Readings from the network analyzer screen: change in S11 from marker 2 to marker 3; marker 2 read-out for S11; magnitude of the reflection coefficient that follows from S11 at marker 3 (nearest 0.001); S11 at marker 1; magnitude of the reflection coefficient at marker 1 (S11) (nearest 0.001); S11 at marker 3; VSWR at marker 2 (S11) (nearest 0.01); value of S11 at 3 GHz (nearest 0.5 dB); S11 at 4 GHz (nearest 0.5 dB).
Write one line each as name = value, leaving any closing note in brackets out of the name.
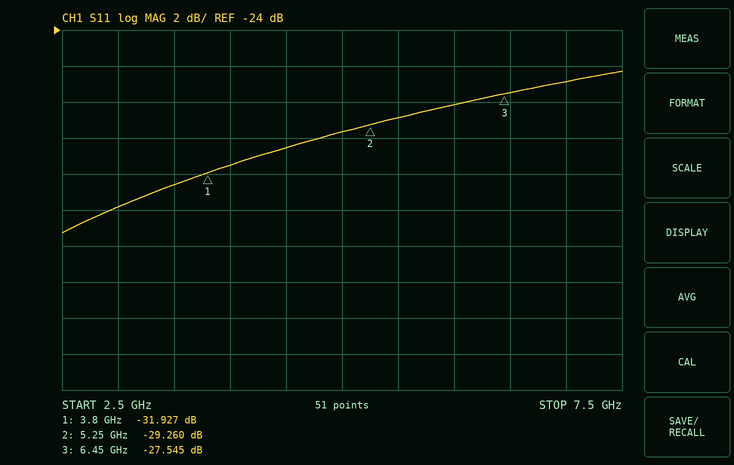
change in S11 from marker 2 to marker 3 = 1.715 dB
marker 2 read-out for S11 = -29.260 dB
magnitude of the reflection coefficient that follows from S11 at marker 3 = 0.042
S11 at marker 1 = -31.927 dB
magnitude of the reflection coefficient at marker 1 (S11) = 0.025
S11 at marker 3 = -27.545 dB
VSWR at marker 2 (S11) = 1.07
value of S11 at 3 GHz = -34.0 dB
S11 at 4 GHz = -31.5 dB
